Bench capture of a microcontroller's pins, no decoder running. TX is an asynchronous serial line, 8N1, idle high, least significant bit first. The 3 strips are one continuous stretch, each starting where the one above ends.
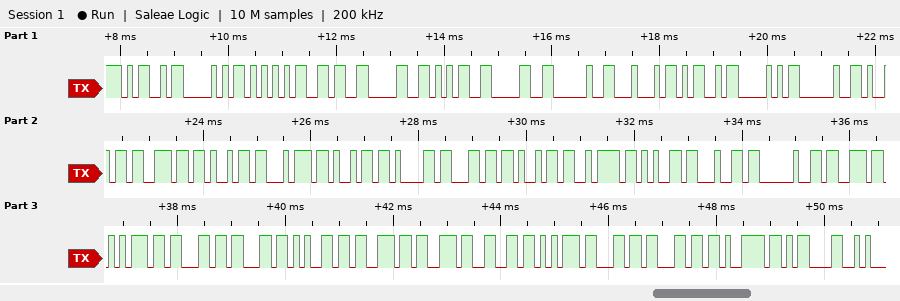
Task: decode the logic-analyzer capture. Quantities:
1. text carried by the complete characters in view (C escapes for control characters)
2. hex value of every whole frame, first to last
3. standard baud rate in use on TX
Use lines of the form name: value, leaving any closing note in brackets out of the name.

text carried by the complete characters in view: "MPU6050 DMP initialized successfully\r"
hex value of every whole frame, first to last: 4D 50 55 36 30 35 30 20 44 4D 50 20 69 6E 69 74 69 61 6C 69 7A 65 64 20 73 75 63 63 65 73 73 66 75 6C 6C 79 0D
standard baud rate in use on TX: 9600 baud
